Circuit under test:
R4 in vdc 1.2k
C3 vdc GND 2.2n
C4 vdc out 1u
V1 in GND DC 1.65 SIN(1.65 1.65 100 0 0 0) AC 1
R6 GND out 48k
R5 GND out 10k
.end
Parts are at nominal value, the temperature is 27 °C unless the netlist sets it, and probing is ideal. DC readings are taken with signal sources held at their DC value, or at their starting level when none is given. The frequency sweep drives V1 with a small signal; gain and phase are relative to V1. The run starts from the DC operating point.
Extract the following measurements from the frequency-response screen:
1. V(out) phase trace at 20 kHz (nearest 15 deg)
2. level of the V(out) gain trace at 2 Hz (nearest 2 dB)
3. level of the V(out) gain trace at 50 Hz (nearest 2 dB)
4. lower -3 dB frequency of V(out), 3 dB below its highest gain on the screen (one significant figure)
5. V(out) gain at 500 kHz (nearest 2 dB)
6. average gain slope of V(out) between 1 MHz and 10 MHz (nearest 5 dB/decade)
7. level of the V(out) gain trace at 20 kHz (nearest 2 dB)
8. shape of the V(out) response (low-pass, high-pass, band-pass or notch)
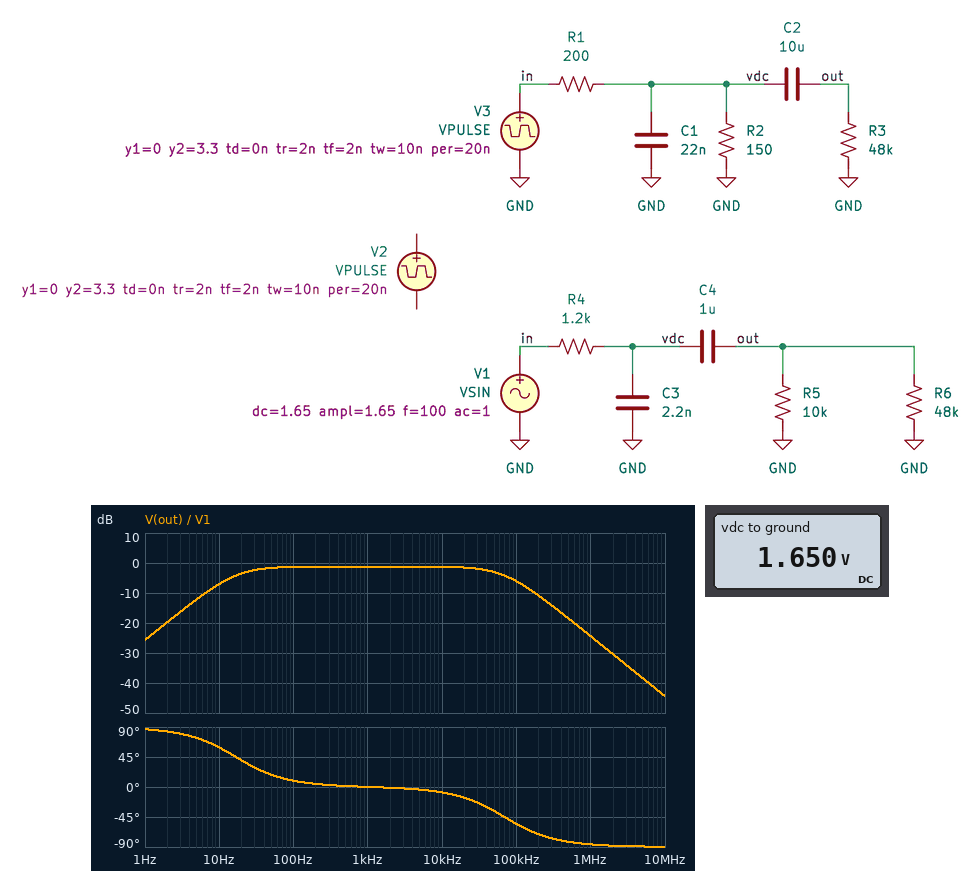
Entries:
-15 deg
-20 dB
-2 dB
20 Hz
-18 dB
-20 dB/decade
-2 dB
band-pass
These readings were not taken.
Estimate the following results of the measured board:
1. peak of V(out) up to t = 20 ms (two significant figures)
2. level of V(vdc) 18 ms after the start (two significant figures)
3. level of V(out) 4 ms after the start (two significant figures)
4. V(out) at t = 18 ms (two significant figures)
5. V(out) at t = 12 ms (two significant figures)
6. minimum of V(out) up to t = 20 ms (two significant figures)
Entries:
1.4 V
270 mV
480 mV
-1.3 V
1.3 V
-1.5 V
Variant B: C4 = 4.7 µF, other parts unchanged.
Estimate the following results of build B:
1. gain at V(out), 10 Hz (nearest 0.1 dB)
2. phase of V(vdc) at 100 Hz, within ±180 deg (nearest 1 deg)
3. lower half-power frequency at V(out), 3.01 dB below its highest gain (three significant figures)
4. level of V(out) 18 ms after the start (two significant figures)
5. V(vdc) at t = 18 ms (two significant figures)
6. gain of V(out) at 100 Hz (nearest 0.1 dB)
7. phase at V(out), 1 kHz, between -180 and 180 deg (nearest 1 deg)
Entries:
-1.7 dB
0 deg
3.57 Hz
-1.4 V
280 mV
-1.2 dB
-1 deg
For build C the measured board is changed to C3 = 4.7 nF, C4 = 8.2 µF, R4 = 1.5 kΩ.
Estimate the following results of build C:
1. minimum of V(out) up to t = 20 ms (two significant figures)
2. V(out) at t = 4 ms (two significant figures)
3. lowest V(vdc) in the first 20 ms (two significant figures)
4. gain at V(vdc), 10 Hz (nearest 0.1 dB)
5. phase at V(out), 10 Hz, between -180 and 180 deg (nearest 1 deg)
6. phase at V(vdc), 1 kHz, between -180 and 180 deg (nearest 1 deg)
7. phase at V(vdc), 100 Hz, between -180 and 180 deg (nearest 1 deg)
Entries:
-1.4 V
780 mV
260 mV
-1.4 dB
11 deg
-2 deg
0 deg
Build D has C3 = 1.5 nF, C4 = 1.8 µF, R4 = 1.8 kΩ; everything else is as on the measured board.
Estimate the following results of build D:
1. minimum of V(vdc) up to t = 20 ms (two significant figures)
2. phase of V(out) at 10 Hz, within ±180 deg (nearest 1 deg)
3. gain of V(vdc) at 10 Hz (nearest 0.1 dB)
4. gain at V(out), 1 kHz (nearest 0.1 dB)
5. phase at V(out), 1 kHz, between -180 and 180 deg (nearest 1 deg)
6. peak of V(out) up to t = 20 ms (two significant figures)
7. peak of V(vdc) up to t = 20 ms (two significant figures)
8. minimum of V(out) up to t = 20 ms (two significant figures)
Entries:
300 mV
41 deg
-0.9 dB
-1.7 dB
0 deg
1.3 V
3.0 V
-1.4 V
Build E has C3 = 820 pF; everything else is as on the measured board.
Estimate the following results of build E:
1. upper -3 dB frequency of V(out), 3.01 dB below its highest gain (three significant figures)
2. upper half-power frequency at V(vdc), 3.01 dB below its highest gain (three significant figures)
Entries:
185 kHz
134 kHz
